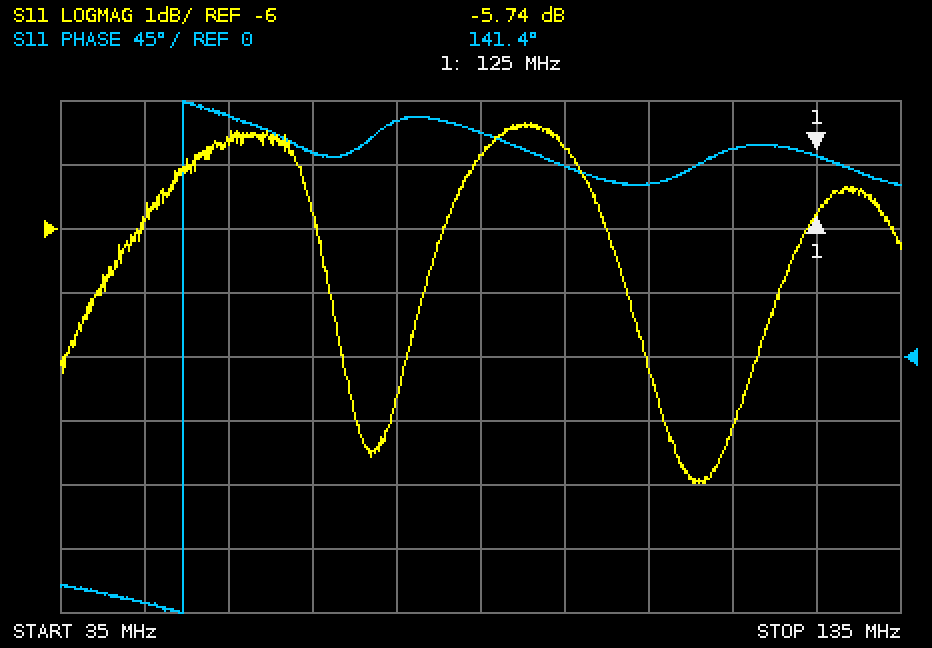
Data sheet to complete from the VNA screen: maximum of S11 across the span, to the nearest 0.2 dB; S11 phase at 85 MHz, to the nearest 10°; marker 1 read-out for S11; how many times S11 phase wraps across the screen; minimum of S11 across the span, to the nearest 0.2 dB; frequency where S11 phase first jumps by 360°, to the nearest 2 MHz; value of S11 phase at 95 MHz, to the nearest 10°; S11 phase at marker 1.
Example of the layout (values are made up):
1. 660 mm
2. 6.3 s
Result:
1. -4.4 dB
2. 160°
3. -5.74 dB
4. 1
5. -10.0 dB
6. 50 MHz
7. 130°
8. 141.4°
